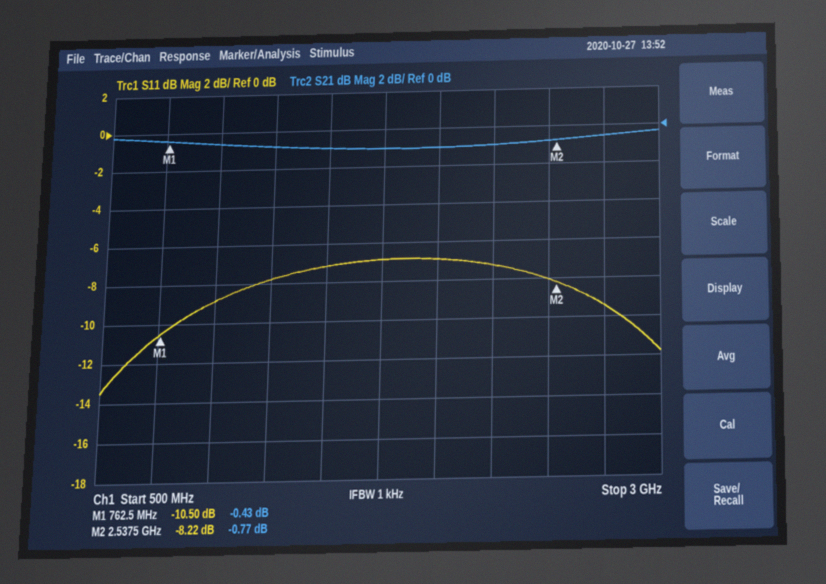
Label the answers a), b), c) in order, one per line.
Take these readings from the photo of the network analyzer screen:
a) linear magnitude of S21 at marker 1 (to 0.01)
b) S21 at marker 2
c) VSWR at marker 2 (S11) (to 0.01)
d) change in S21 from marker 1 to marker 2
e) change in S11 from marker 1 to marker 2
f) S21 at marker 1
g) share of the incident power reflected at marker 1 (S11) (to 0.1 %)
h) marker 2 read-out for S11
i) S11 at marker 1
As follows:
a) 0.95
b) -0.77 dB
c) 2.27
d) -0.34 dB
e) 2.28 dB
f) -0.43 dB
g) 8.9 %
h) -8.22 dB
i) -10.50 dB
